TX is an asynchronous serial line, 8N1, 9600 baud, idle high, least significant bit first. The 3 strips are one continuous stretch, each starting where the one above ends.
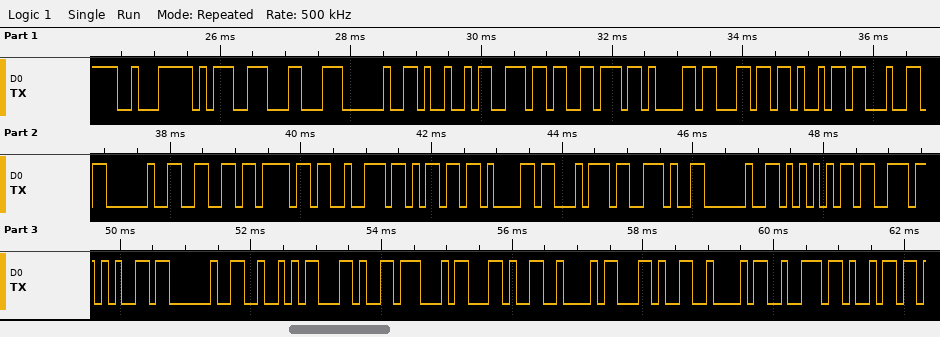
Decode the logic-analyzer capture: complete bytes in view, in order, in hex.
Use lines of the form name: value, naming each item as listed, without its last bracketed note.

complete bytes in view, in order, in hex: E2 9D 8C 20 49 6E 76 61 6C 69 64 20 66 6F 72 6D 61 74 2E 20 55 73 65 20 52 2C 47 2C 42 2C 42 72 69
